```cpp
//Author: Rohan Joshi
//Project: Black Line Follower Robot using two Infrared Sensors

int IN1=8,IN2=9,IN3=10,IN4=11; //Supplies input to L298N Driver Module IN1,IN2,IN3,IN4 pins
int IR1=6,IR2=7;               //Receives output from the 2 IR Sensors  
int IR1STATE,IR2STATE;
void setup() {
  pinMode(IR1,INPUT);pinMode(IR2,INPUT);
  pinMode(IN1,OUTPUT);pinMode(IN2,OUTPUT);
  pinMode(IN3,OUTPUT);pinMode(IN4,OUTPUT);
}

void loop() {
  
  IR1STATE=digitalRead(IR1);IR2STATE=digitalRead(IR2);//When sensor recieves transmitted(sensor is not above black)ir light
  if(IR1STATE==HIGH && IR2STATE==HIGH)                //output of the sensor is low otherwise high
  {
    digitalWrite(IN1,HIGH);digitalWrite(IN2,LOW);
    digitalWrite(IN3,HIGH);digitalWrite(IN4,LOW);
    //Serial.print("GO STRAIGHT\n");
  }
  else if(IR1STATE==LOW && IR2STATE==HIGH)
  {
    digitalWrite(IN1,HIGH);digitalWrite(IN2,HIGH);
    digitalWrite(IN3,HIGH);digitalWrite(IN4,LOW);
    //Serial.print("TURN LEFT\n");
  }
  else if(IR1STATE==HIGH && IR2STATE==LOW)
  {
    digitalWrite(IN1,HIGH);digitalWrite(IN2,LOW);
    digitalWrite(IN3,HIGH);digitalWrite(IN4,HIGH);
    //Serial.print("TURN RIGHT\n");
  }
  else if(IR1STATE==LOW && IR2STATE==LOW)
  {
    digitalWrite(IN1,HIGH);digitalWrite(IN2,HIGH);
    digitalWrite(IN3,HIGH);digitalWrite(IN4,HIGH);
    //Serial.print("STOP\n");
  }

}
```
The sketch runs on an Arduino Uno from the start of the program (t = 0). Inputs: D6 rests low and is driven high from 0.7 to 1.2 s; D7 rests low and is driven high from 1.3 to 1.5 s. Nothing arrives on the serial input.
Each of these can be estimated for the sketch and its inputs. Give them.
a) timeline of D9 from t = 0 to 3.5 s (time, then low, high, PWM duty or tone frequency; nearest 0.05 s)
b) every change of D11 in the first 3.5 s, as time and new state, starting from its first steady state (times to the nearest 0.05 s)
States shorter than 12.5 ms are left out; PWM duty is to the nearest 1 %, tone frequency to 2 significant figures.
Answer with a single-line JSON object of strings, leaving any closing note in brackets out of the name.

{"timeline of D9 from t = 0 to 3.5 s": "0 s high; 0.7 s low; 1.2 s high", "every change of D11 in the first 3.5 s, as time and new state, starting from its first steady state": "0 s high; 1.3 s low; 1.5 s high"}
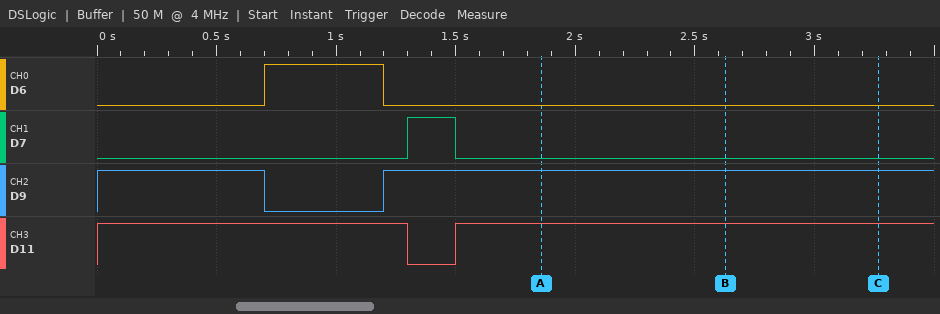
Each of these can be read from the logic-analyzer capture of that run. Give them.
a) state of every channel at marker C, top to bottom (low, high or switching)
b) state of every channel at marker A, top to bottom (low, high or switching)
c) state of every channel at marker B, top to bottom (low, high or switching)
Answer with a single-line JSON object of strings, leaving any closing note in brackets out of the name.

{"state of every channel at marker C, top to bottom": "D6 low, D7 low, D9 high, D11 high", "state of every channel at marker A, top to bottom": "D6 low, D7 low, D9 high, D11 high", "state of every channel at marker B, top to bottom": "D6 low, D7 low, D9 high, D11 high"}
